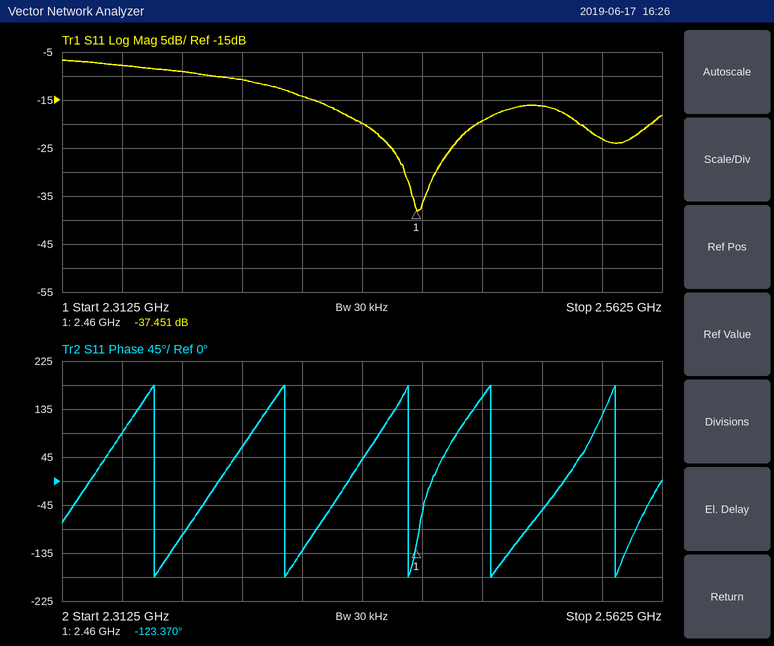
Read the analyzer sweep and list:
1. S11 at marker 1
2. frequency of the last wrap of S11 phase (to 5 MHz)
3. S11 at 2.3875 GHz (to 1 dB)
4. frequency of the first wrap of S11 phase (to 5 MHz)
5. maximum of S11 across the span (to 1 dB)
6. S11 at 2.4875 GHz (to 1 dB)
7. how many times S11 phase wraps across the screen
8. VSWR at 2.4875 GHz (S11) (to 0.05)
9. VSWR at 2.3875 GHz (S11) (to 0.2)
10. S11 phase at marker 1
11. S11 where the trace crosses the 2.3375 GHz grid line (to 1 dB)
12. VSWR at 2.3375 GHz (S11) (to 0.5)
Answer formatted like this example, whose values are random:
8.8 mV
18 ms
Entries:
-37.451 dB
2.545 GHz
-11 dB
2.350 GHz
-7 dB
-19 dB
5
1.25
1.8
-123.370°
-8 dB
2.5
